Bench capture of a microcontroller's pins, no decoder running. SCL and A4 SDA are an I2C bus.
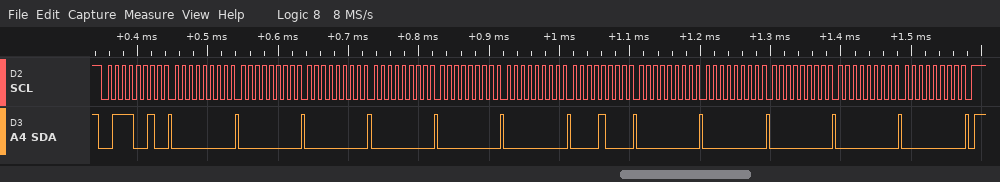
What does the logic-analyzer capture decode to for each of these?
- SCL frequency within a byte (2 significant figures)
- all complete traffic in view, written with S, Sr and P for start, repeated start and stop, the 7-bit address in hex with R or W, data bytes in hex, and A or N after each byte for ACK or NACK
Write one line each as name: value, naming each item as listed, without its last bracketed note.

SCL frequency within a byte: 100 kHz
all complete traffic in view, written with S, Sr and P for start, repeated start and stop, the 7-bit address in hex with R or W, data bytes in hex, and A or N after each byte for ACK or NACK: S 39W A 00 A 00 A 00 A 00 A 00 A 00 A 08 A 00 A 00 A 00 A 00 A 00 A P
